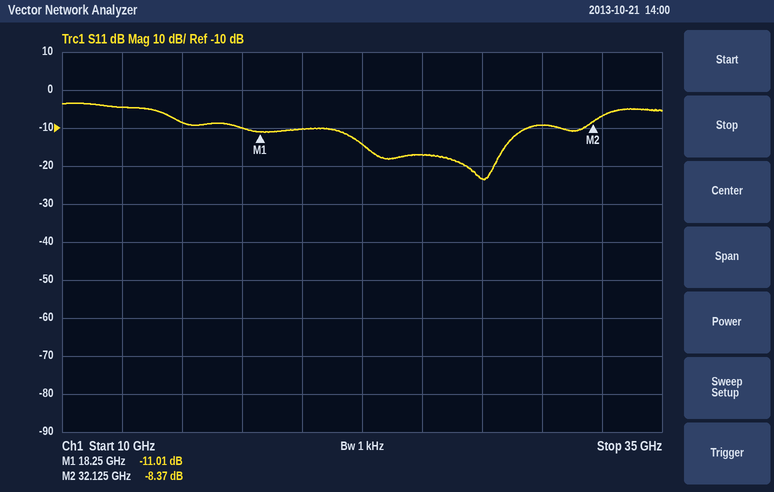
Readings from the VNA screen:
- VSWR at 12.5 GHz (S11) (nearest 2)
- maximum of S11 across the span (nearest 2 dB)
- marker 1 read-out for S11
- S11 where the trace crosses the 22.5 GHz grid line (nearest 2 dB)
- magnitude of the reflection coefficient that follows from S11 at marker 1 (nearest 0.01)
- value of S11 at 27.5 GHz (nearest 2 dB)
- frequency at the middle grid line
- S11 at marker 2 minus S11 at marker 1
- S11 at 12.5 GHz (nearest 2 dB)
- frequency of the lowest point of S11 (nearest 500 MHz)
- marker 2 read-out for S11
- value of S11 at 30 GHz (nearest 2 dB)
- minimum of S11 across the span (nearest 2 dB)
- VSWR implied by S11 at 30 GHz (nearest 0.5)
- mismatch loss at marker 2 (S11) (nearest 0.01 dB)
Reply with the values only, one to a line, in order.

4
-4 dB
-11.01 dB
-14 dB
0.28
-24 dB
22.5 GHz
2.64 dB
-4 dB
27.5 GHz
-8.37 dB
-10 dB
-24 dB
2.0
0.68 dB
